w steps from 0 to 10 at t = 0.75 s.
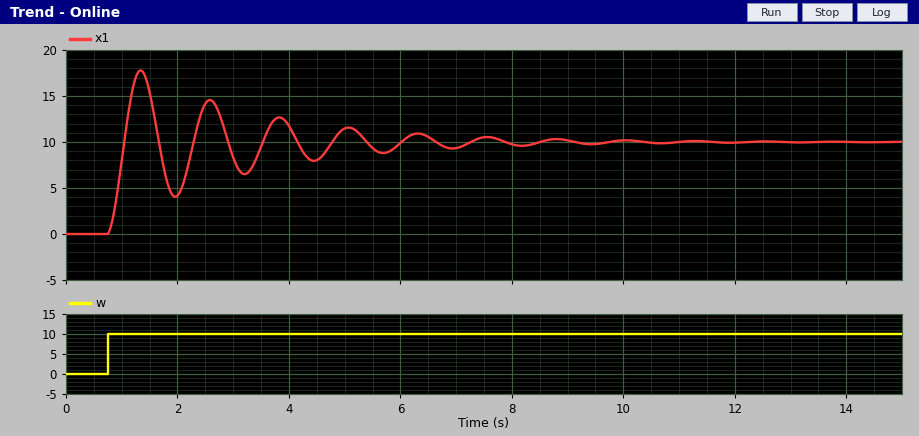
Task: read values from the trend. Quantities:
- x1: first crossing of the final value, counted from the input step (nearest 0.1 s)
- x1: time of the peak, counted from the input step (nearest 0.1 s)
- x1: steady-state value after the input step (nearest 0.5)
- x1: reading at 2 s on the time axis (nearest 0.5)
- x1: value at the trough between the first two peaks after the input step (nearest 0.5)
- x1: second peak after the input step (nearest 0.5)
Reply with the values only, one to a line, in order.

0.3 s
0.6 s
10.0
4.0
4.0
14.5
